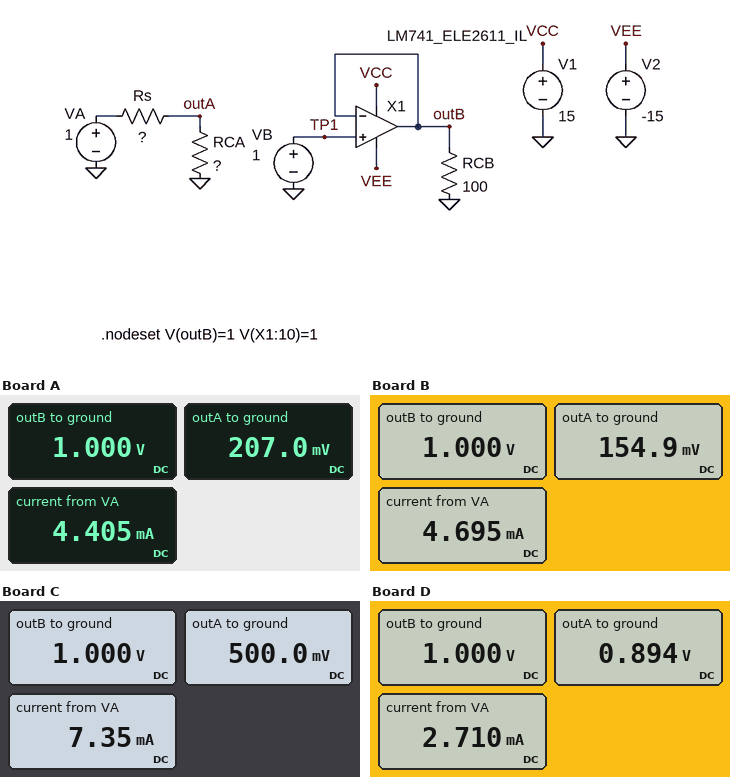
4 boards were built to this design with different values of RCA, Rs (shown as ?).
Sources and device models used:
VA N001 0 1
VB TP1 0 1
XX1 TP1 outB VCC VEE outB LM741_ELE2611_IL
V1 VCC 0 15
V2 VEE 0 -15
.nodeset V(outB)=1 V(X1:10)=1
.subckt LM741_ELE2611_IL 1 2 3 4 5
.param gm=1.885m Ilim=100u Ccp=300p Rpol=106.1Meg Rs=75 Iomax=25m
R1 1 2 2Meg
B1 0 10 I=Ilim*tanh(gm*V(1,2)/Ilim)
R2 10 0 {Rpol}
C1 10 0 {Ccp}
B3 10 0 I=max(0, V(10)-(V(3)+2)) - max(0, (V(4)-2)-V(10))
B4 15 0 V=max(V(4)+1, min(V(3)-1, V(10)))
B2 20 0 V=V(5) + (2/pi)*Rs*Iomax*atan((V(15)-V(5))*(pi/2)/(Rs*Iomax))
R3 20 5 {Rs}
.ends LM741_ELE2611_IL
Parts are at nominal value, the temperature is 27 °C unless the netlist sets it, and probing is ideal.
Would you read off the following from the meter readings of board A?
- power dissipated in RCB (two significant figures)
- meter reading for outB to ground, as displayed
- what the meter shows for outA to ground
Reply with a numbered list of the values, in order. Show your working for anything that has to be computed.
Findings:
1. (1 V)^2 / 100 Ω = 10 mW
2. 1.000 V
3. 207.0 mV
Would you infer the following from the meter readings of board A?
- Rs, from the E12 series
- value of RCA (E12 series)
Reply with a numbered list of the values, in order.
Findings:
1. 180 Ω
2. 47 Ω
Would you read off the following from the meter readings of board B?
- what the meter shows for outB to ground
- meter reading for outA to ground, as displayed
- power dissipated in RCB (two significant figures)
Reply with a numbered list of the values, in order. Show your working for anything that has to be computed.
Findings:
1. 1.000 V
2. 154.9 mV
3. (1 V)^2 / 100 Ω = 10 mW
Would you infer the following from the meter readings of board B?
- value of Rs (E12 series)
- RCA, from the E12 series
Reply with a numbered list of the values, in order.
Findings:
1. 180 Ω
2. 33 Ω
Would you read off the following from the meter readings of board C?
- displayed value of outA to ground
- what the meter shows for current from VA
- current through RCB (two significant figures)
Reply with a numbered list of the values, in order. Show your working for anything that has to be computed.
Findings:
1. 500.0 mV
2. 7.35 mA
3. (1 V) / 100 Ω = 10 mA
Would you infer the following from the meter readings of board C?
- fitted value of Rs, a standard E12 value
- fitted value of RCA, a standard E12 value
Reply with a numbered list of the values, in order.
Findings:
1. 68 Ω
2. 68 Ω
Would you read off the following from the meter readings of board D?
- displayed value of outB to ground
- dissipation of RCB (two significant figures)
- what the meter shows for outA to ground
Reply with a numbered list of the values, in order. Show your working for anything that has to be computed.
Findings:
1. 1.000 V
2. (1 V)^2 / 100 Ω = 10 mW
3. 0.894 V
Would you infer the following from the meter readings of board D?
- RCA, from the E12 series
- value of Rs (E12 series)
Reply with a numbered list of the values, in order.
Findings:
1. 330 Ω
2. 39 Ω
